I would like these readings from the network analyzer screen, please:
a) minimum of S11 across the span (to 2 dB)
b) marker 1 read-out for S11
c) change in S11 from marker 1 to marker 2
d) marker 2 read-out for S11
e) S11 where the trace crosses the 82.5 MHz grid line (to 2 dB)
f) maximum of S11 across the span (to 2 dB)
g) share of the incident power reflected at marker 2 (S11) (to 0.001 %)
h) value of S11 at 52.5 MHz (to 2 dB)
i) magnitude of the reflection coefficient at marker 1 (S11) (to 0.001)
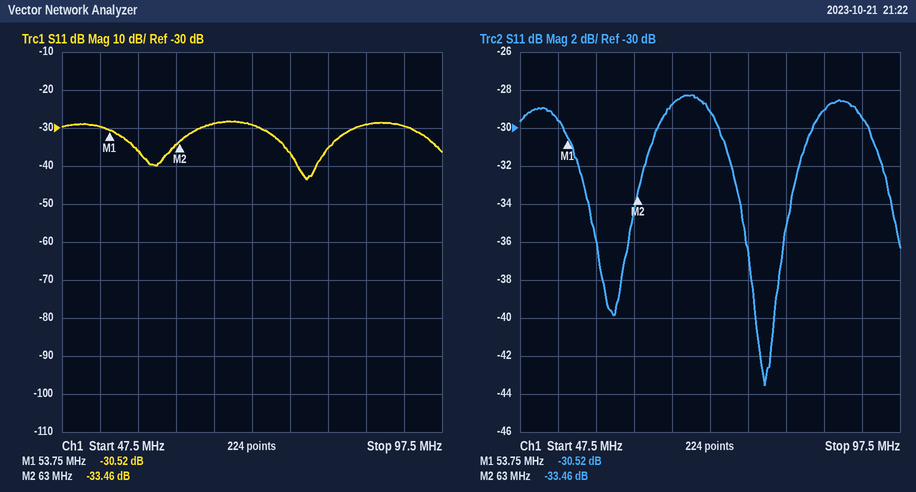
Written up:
-44 dB
-30.52 dB
-2.94 dB
-33.46 dB
-36 dB
-28 dB
0.045 %
-30 dB
0.030
